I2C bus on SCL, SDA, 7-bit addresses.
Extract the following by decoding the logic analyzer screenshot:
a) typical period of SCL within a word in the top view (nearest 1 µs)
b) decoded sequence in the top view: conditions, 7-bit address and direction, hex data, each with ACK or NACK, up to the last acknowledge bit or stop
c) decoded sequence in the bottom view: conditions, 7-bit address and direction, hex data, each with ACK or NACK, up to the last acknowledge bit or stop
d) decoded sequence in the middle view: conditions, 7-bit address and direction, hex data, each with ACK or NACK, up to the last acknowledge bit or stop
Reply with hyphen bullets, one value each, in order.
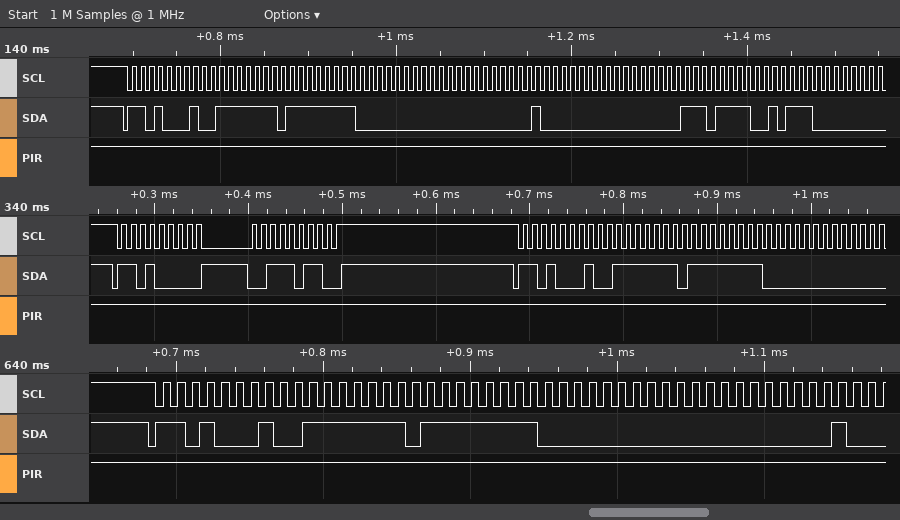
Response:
- 10 µs
- start, address 68 read ACK, 7F ACK, FF ACK, 00 ACK, 00 ACK, 40 ACK, 00 ACK, EF ACK, 5C ACK
- start, address 68 read ACK, 7F ACK, FF ACK, 00 ACK, 00 ACK
- start, address 68 write ACK, 3B ACK, stop, start, address 68 read ACK, 7F ACK, FF ACK, 00 ACK
